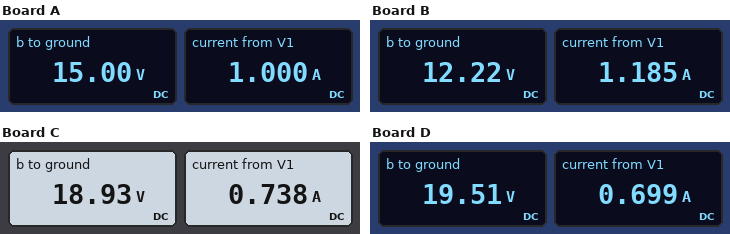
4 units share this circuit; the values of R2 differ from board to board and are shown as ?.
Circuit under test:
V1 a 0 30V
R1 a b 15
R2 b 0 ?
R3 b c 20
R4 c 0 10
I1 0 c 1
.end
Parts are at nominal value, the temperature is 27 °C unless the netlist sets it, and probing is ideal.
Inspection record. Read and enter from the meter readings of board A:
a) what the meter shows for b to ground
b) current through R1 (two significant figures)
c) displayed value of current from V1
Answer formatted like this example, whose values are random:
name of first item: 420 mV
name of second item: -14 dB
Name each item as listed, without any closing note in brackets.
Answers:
what the meter shows for b to ground: 15.00 V
current through R1: 1.0 A
displayed value of current from V1: 1.000 A
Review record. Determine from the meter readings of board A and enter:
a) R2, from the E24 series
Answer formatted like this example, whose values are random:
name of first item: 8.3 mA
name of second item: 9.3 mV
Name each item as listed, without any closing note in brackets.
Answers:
R2, from the E24 series: 18 Ω
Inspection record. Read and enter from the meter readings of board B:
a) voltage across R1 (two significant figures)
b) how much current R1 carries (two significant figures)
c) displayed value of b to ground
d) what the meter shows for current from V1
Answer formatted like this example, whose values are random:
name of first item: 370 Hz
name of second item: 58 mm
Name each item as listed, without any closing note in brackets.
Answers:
voltage across R1: 18 V
how much current R1 carries: 1.2 A
displayed value of b to ground: 12.22 V
what the meter shows for current from V1: 1.185 A
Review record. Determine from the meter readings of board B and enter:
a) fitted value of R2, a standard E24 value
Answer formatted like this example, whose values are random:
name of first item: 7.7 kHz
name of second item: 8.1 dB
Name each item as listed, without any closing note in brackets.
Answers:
fitted value of R2, a standard E24 value: 11 Ω
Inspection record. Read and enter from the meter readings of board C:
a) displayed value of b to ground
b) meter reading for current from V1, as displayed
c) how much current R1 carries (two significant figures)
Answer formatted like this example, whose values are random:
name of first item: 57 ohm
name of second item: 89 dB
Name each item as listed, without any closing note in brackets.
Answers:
displayed value of b to ground: 18.93 V
meter reading for current from V1, as displayed: 0.738 A
how much current R1 carries: 740 mA
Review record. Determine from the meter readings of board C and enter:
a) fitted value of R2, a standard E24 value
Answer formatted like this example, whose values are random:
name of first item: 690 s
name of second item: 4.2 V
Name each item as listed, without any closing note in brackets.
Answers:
fitted value of R2, a standard E24 value: 43 Ω
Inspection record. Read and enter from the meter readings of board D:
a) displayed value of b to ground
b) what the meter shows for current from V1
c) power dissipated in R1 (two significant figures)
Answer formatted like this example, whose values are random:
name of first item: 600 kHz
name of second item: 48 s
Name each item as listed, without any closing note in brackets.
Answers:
displayed value of b to ground: 19.51 V
what the meter shows for current from V1: 0.699 A
power dissipated in R1: 7.3 W
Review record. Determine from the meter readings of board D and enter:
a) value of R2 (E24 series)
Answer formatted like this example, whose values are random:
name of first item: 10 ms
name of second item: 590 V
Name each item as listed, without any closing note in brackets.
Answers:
value of R2: 51 Ω
